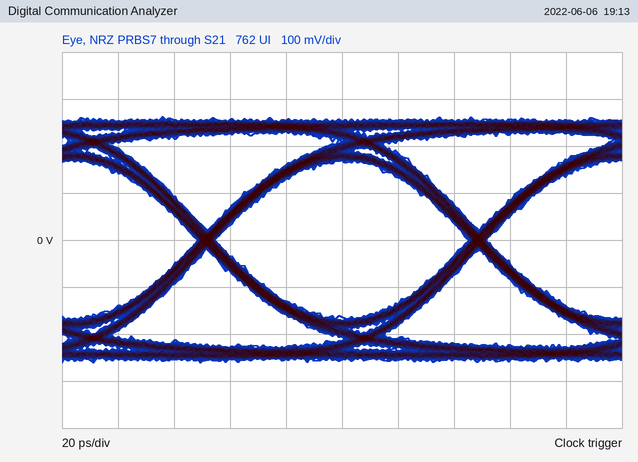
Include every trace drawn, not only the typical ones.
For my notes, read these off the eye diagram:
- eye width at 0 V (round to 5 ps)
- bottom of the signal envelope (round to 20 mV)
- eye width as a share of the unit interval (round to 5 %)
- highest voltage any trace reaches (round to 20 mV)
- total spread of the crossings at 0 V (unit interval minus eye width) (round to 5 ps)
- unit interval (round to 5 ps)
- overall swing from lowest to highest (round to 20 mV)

90 ps
-260 mV
95 %
260 mV
5 ps
95 ps
520 mV
